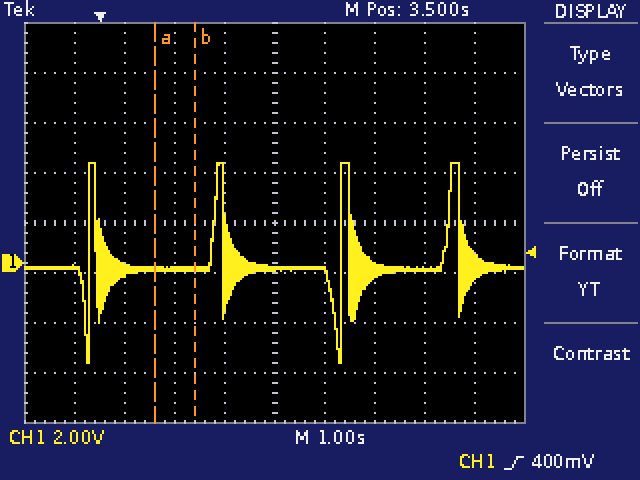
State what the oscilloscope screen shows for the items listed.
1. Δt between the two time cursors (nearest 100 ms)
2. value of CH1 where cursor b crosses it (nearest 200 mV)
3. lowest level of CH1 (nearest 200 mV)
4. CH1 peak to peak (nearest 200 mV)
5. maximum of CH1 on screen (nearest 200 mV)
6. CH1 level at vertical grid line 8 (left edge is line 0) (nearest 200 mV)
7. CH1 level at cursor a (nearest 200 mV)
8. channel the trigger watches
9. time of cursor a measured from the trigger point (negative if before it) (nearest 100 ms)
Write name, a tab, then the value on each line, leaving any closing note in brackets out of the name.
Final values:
Δt between the two time cursors	800 ms
value of CH1 where cursor b crosses it	-200 mV
lowest level of CH1	-4.0 V
CH1 peak to peak	8.0 V
maximum of CH1 on screen	4.0 V
CH1 level at vertical grid line 8 (left edge is line 0)	-200 mV
CH1 level at cursor a	-200 mV
channel the trigger watches	CH1
time of cursor a measured from the trigger point (negative if before it)	+1.1 s
